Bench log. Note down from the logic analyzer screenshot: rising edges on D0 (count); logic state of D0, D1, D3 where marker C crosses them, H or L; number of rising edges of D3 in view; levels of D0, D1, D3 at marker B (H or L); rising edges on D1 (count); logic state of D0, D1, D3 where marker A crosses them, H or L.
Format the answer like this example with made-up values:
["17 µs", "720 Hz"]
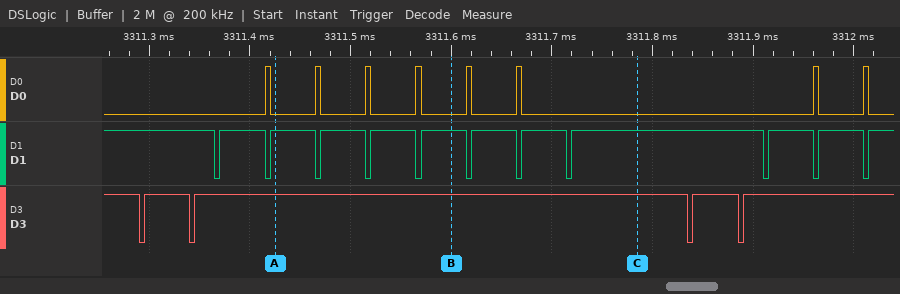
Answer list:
["8", "D0=L, D1=H, D3=H", "4", "D0=L, D1=H, D3=H", "11", "D0=L, D1=H, D3=H"]
